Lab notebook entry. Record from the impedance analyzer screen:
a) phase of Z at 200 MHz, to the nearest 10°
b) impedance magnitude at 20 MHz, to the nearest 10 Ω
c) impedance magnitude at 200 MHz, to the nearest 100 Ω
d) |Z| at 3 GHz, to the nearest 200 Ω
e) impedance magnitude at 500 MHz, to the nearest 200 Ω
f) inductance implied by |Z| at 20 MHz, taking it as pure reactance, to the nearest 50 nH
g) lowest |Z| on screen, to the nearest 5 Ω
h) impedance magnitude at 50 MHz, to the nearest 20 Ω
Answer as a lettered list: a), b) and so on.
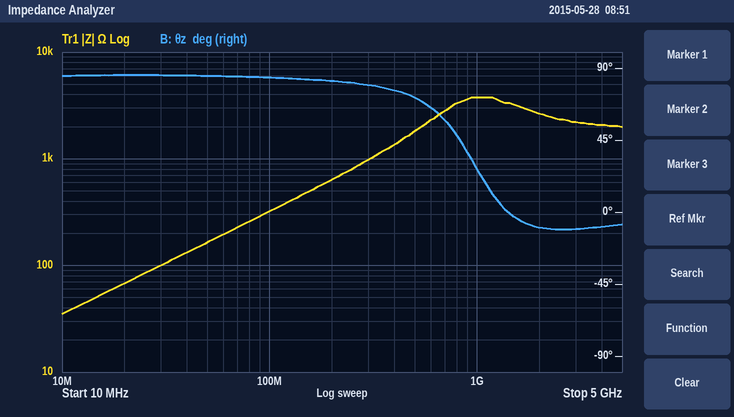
a) 80°
b) 70 Ω
c) 600 Ω
d) 2.2 kΩ
e) 1.8 kΩ
f) 550 nH
g) 35 Ω
h) 160 Ω
